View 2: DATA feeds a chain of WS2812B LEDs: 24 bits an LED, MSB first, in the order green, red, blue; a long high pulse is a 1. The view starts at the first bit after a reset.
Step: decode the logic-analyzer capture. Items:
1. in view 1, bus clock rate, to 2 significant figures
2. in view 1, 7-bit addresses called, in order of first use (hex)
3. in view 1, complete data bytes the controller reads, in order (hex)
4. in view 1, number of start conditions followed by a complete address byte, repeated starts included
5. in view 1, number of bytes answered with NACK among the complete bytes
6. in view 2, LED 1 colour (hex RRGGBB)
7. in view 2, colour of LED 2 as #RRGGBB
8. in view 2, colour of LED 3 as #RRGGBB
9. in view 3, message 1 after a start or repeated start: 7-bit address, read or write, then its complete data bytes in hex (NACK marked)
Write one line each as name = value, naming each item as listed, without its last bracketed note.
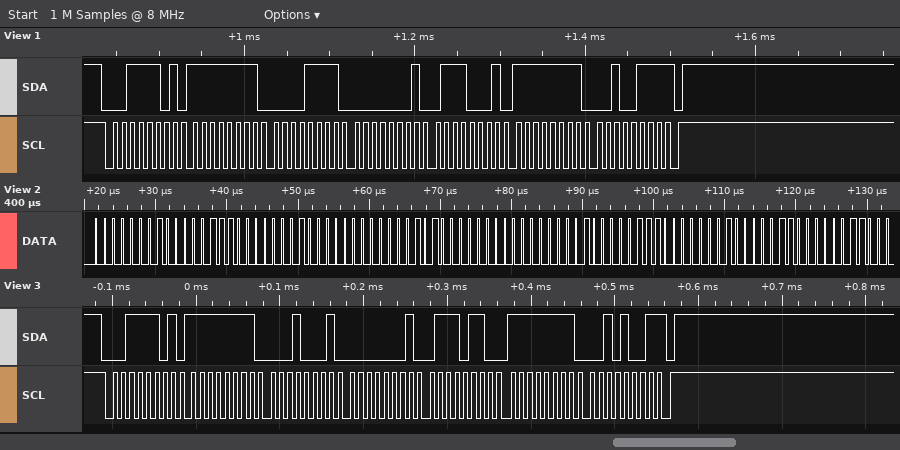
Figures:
in view 1, bus clock rate, to 2 significant figures = 100 kHz
in view 1, 7-bit addresses called, in order of first use = 0x1E
in view 1, complete data bytes the controller reads, in order = FF 0F 01 71 FF 27
in view 1, number of start conditions followed by a complete address byte, repeated starts included = 1
in view 1, number of bytes answered with NACK among the complete bytes = 1
in view 2, LED 1 colour = #070101
in view 2, colour of LED 2 as #RRGGBB = #0A0000
in view 2, colour of LED 3 as #RRGGBB = #070101
in view 3, message 1 after a start or repeated start: 7-bit address, read or write, then its complete data bytes in hex = 0x1E read: FF 11 01 76 FF 29 NACK
